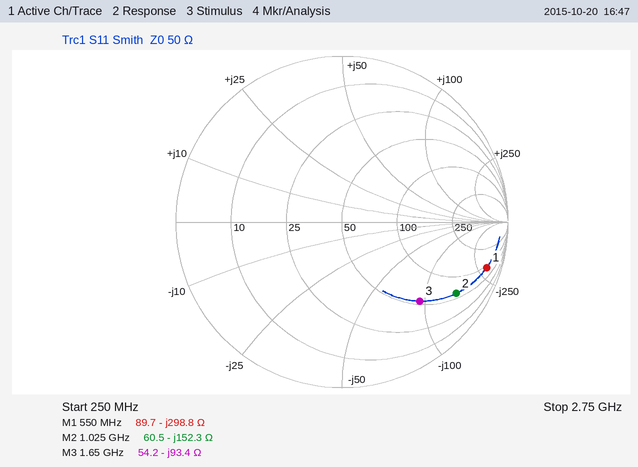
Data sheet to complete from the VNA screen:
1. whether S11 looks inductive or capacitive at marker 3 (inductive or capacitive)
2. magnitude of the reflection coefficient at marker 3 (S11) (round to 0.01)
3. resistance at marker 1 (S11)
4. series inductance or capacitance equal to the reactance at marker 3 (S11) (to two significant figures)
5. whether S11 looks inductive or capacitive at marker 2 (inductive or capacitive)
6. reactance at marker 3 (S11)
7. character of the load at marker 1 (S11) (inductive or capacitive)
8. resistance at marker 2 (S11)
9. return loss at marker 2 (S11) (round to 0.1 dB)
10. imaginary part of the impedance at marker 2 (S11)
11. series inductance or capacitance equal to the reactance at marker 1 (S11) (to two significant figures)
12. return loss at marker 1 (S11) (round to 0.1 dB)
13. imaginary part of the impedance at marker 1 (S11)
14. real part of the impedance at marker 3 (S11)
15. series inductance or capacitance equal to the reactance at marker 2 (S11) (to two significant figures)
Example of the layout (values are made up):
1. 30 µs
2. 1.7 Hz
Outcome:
1. capacitive
2. 0.67
3. 89.7 Ω
4. 1.0 pF
5. capacitive
6. -93.4 Ω
7. capacitive
8. 60.5 Ω
9. 1.8 dB
10. -152.3 Ω
11. 970 fF
12. 0.8 dB
13. -298.8 Ω
14. 54.2 Ω
15. 1.0 pF
